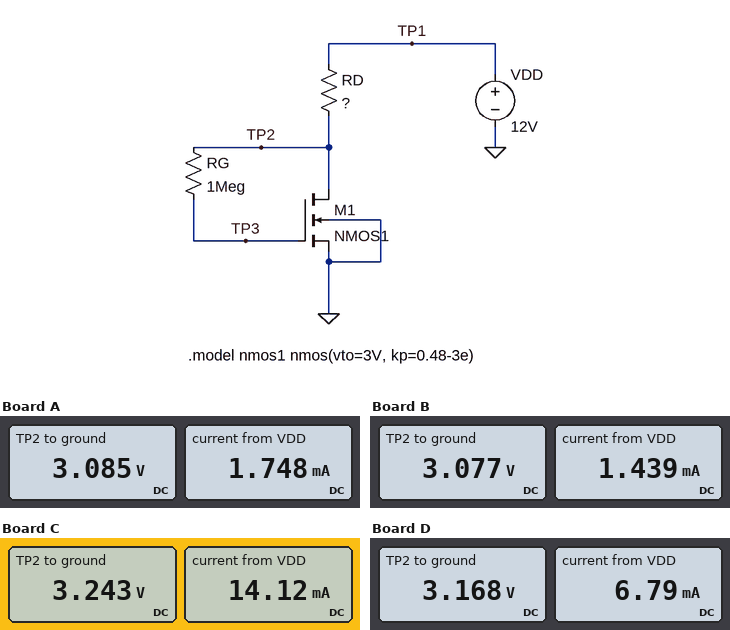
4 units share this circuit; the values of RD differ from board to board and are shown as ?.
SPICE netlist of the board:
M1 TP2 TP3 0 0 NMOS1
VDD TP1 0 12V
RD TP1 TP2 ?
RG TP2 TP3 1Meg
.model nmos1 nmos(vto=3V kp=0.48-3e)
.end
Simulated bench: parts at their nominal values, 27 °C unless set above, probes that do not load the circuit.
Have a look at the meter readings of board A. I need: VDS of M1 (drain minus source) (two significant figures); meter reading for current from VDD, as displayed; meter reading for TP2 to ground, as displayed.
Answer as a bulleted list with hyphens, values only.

- 3.1 V
- 1.748 mA
- 3.085 V
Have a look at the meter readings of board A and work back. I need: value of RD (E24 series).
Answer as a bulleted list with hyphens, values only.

- 5.1 kΩ
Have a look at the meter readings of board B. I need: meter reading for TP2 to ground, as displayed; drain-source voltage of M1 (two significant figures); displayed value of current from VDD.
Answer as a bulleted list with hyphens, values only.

- 3.077 V
- 3.1 V
- 1.439 mA
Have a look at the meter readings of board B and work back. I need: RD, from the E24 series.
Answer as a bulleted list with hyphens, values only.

- 6.2 kΩ
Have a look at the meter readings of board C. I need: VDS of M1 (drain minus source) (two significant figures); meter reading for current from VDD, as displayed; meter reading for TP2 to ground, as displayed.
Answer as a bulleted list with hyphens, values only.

- 3.2 V
- 14.12 mA
- 3.243 V
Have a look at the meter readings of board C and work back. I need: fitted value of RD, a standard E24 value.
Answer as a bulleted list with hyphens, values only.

- 620 Ω
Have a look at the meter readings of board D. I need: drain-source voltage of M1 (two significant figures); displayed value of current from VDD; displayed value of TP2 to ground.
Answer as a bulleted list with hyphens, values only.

- 3.2 V
- 6.79 mA
- 3.168 V
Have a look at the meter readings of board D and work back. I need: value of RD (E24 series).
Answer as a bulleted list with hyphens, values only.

- 1.3 kΩ
